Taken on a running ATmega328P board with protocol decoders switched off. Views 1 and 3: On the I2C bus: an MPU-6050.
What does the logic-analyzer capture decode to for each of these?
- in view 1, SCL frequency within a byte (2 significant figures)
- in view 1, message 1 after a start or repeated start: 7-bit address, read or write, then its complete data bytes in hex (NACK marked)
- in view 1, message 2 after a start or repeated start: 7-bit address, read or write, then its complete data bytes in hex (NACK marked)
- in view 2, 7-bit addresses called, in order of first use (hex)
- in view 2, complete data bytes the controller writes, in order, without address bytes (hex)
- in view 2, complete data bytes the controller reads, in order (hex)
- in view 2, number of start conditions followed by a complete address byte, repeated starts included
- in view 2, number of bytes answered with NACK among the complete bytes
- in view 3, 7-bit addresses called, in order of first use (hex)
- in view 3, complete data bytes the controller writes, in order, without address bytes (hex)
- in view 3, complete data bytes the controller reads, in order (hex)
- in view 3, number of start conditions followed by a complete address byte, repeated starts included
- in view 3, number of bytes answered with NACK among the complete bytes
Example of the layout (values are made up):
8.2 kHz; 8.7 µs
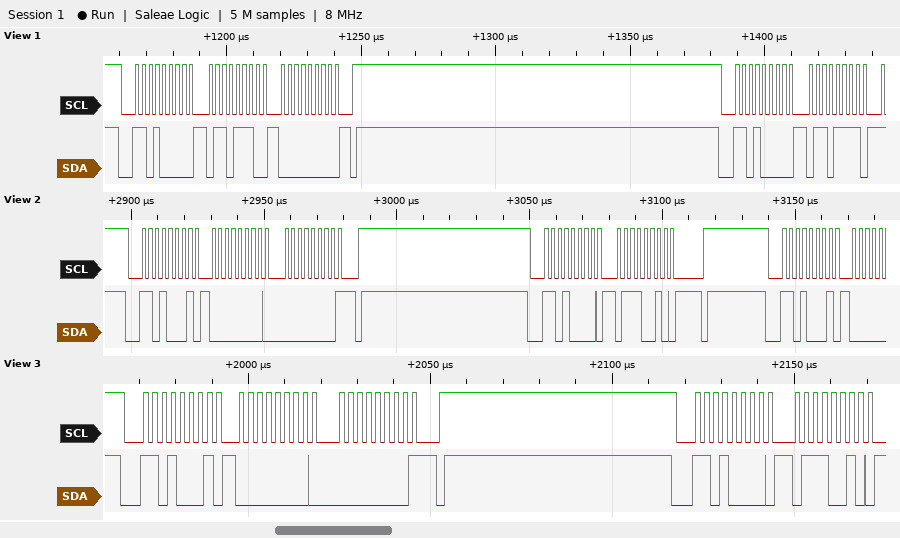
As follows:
400 kHz; 0x68 write: 6E 00; 0x68 write: 6F; 0x68; 72; 00 00; 3; 1; 0x68; 72; 00 00; 2; 1
